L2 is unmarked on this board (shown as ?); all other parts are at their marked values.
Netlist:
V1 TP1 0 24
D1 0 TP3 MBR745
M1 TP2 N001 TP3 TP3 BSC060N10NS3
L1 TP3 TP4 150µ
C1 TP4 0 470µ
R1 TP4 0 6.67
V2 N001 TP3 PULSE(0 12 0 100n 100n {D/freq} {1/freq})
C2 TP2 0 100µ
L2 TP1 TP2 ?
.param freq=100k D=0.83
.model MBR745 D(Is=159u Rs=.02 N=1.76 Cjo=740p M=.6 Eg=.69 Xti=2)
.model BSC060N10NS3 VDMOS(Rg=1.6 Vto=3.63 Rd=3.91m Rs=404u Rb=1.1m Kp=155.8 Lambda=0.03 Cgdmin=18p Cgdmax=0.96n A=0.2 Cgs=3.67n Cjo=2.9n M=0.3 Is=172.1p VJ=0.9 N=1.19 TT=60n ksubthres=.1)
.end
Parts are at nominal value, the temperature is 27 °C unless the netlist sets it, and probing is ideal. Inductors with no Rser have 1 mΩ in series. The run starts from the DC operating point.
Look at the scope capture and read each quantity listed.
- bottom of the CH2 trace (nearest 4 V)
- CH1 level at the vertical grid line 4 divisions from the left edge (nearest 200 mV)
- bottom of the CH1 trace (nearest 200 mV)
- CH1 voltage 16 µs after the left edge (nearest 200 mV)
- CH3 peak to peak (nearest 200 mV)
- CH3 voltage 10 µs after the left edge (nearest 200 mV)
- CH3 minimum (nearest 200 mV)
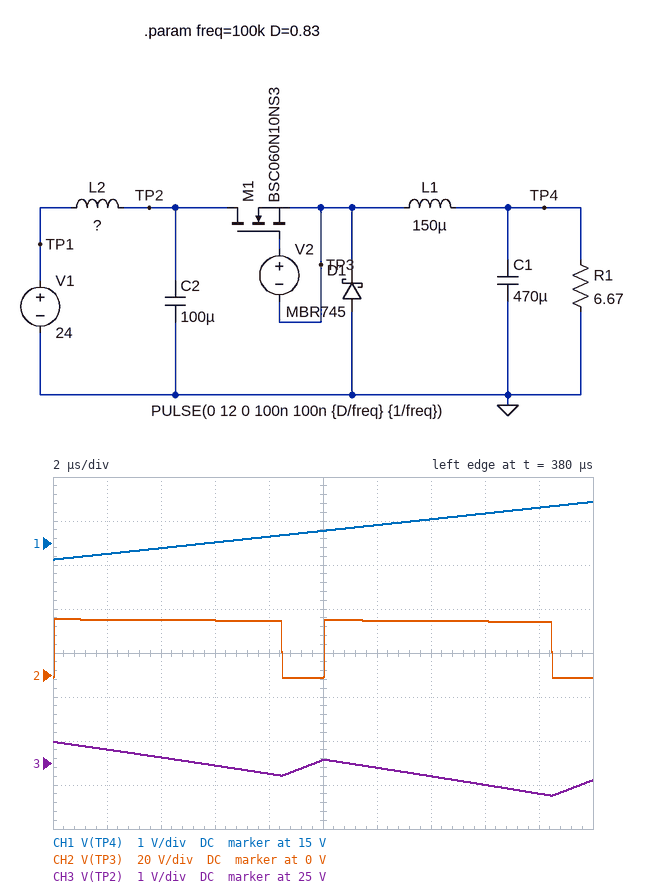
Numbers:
0 V
15.2 V
14.6 V
15.6 V
1.2 V
25.0 V
24.2 V
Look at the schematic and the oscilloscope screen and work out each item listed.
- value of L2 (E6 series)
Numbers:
33 µH
